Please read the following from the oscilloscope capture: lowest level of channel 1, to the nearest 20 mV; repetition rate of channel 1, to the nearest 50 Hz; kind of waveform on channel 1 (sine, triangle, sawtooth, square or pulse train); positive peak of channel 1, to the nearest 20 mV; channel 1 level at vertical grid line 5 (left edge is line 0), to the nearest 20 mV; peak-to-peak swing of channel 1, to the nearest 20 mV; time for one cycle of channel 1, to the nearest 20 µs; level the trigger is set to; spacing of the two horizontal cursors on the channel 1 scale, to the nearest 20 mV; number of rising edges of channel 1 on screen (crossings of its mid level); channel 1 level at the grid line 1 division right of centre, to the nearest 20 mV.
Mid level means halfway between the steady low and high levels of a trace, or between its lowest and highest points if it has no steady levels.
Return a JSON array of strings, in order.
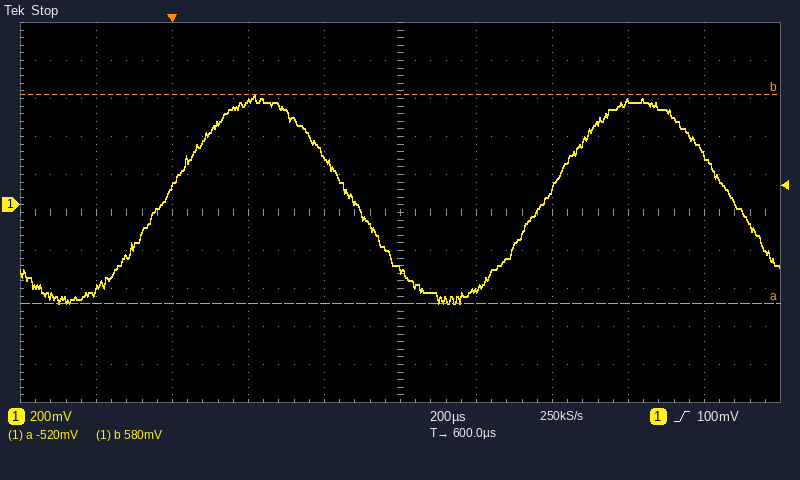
["-520 mV", "1.00 kHz", "sine", "580 mV", "-340 mV", "1.10 V", "1.00 ms", "100 mV", "1.10 V", "2", "-440 mV"]
